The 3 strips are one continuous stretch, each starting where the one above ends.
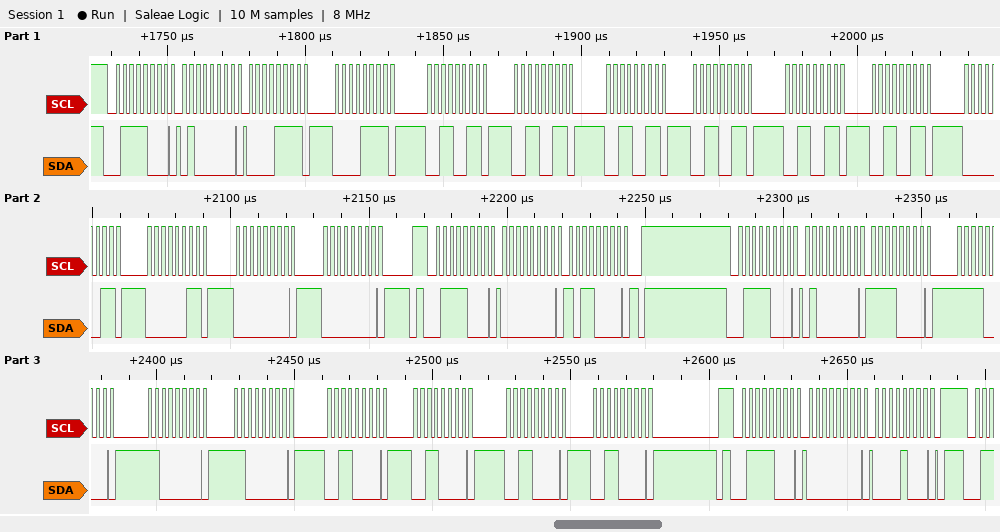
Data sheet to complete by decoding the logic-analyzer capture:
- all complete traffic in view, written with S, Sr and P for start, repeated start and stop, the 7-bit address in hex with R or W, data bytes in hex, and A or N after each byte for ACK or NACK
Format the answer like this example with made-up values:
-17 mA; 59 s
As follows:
S 3CW A 40 A 0F A 0F A 33 A 33 A 33 A 33 A 33 A 33 A 03 A 03 A 00 A 00 A P S 3CW A 00 A B0 A P S 3CW A 40 A F0 A F0 A C0 A C0 A 30 A 30 A 30 A 30 A P S 3CW A 00 A 08 A P
